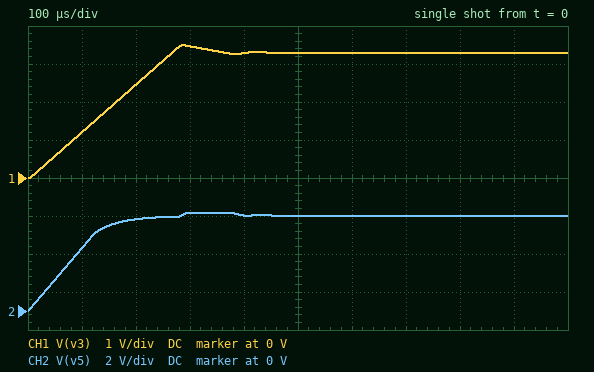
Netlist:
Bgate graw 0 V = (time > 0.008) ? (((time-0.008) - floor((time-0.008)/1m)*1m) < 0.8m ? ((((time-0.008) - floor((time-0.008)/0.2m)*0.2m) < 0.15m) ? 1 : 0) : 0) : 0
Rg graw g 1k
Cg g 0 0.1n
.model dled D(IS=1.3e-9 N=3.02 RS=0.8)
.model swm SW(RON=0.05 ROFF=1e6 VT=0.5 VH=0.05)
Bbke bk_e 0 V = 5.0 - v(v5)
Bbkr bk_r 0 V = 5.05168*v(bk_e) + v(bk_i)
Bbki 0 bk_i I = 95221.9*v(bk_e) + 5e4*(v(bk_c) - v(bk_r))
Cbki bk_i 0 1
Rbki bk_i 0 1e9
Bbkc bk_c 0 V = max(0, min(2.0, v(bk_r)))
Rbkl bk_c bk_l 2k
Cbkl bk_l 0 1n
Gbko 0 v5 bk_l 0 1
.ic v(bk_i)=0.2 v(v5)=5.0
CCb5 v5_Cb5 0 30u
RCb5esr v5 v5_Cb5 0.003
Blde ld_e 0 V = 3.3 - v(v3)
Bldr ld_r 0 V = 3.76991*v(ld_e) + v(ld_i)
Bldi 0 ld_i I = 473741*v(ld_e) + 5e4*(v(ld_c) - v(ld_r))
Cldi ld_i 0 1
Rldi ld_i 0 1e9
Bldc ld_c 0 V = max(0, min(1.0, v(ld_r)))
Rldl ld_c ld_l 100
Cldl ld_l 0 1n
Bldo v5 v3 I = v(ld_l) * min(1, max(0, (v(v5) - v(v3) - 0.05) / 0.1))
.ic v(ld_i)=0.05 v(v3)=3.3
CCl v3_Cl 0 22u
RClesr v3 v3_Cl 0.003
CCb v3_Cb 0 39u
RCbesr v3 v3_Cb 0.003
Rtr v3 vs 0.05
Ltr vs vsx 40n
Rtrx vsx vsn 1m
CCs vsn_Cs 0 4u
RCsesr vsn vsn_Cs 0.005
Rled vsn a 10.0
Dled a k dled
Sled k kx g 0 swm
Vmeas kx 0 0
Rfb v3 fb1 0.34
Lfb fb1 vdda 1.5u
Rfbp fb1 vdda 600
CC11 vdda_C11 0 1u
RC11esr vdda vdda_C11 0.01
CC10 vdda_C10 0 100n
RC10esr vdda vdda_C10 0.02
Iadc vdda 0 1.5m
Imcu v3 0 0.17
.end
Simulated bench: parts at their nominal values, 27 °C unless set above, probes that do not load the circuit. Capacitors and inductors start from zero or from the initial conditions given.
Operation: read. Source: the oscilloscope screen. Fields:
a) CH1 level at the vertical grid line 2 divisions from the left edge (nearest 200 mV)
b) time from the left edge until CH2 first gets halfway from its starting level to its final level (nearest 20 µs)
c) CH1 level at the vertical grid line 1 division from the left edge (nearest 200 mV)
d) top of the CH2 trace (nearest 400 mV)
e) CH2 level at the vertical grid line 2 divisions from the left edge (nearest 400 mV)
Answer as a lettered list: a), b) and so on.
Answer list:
a) 2.4 V
b) 80 µs
c) 1.2 V
d) 5.2 V
e) 4.8 V
